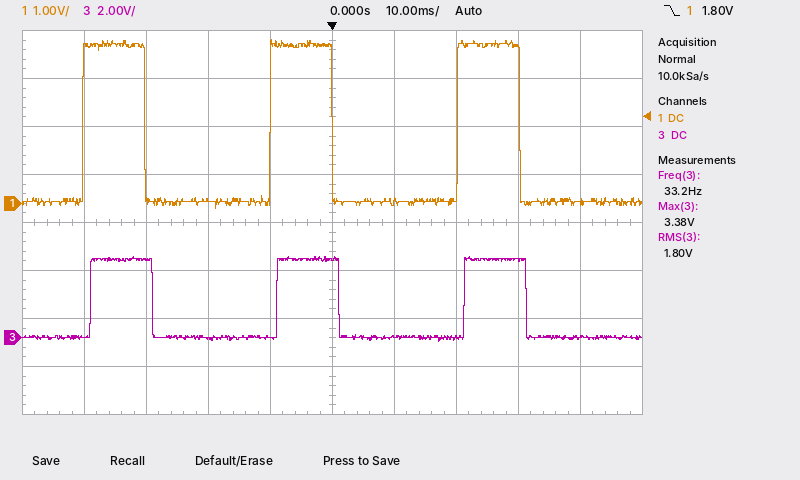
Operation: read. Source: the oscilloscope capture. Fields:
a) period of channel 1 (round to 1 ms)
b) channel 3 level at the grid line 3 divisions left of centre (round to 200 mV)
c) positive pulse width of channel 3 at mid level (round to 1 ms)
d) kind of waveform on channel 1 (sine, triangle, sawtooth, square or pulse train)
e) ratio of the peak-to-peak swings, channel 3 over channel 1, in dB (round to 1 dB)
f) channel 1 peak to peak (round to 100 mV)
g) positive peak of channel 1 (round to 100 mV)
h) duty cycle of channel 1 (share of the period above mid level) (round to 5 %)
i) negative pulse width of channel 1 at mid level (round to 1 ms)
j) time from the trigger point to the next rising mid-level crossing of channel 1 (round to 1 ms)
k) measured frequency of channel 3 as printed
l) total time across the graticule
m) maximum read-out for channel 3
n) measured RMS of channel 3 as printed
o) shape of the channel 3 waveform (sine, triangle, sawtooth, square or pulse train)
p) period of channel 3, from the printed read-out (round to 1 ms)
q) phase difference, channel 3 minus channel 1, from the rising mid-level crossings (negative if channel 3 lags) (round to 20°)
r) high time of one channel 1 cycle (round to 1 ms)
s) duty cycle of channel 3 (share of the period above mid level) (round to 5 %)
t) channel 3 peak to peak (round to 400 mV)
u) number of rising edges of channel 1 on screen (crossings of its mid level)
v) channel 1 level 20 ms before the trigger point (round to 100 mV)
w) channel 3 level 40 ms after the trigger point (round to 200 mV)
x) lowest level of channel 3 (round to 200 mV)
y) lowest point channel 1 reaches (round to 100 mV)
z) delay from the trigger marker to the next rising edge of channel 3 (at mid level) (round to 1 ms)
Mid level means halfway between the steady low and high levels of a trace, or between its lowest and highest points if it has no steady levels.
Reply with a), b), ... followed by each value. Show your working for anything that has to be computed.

a) 30 ms
b) 3.2 V
c) 10 ms
d) pulse train
e) 20 log10(3.6 V / 3.5 V) ≈ 0 dB
f) 3.4 V − (-100 mV) = 3.5 V
g) 3.4 V
h) 10 ms / 30 ms ≈ 33.3 %, so 35 % to the nearest 5 %
i) 20 ms
j) 20 ms
k) 33.2 Hz
l) 100 ms
m) 3.38 V
n) 1.80 V
o) pulse train
p) 1 / 33.2 Hz ≈ 30 ms
q) −360° × (+1 ms) / 30 ms ≈ -12.0°, so -20° to the nearest 20°
r) 10 ms
s) 35 %
t) 3.6 V
u) 3
v) 100 mV
w) 0.0 V
x) -200 mV
y) -100 mV
z) 21 ms
